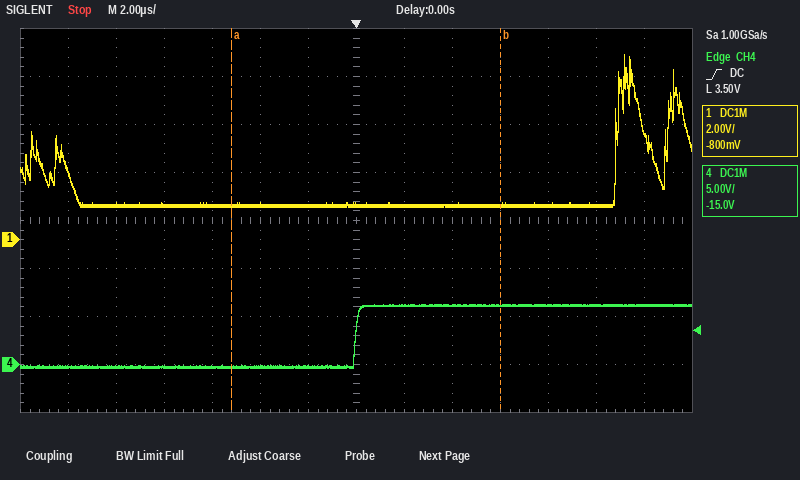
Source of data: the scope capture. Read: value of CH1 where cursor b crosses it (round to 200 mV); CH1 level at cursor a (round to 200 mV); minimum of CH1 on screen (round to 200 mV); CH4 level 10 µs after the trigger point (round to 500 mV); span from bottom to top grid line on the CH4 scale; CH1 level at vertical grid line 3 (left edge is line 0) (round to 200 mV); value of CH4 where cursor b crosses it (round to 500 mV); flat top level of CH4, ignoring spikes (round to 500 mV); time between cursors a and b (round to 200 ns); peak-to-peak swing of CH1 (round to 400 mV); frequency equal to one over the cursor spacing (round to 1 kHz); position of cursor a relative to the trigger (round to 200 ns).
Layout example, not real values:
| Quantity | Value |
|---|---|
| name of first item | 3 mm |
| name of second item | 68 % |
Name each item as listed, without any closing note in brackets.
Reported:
| Quantity | Value |
|---|---|
| value of CH1 where cursor b crosses it | 1.4 V |
| CH1 level at cursor a | 1.4 V |
| minimum of CH1 on screen | 1.4 V |
| CH4 level 10 µs after the trigger point | 6.0 V |
| span from bottom to top grid line on the CH4 scale | 40 V |
| CH1 level at vertical grid line 3 (left edge is line 0) | 1.4 V |
| value of CH4 where cursor b crosses it | 6.0 V |
| flat top level of CH4, ignoring spikes | 6.0 V |
| time between cursors a and b | 11.2 µs |
| peak-to-peak swing of CH1 | 6.4 V |
| frequency equal to one over the cursor spacing | 89 kHz |
| position of cursor a relative to the trigger | -5.2 µs |
